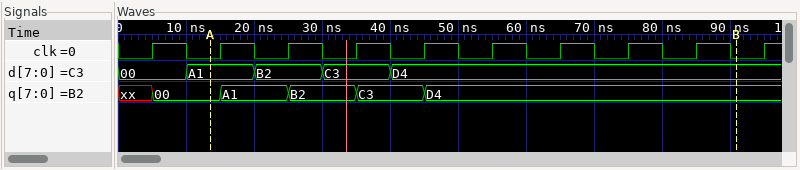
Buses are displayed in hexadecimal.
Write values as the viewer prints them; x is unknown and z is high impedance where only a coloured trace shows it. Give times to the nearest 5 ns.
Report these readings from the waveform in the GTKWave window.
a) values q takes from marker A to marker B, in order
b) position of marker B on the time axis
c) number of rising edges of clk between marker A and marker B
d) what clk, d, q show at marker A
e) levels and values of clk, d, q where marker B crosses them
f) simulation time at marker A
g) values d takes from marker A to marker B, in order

00, A1, B2, C3, D4
90 ns
8
clk=0, d=A1, q=00
clk=0, d=D4, q=D4
15 ns
A1, B2, C3, D4
